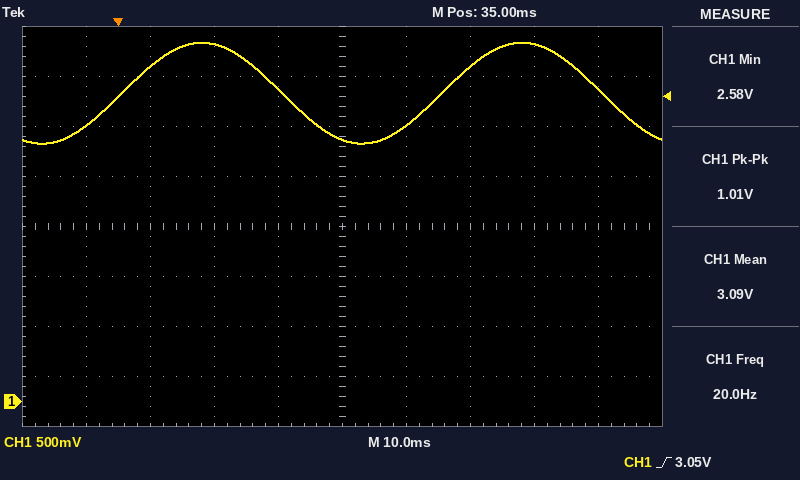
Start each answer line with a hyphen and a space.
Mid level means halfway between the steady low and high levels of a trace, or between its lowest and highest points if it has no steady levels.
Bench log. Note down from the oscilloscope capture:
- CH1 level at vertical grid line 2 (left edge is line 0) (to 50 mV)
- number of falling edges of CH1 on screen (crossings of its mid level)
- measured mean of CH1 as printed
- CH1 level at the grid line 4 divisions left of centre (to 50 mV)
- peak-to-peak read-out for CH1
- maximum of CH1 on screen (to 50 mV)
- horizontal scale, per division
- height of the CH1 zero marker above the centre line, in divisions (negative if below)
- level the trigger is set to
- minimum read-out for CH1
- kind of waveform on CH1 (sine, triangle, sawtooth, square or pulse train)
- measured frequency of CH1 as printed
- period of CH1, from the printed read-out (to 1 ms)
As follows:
- 3.35 V
- 2
- 3.09 V
- 2.75 V
- 1.01 V
- 3.60 V
- 10 ms
- -3.5 div
- 3.05 V
- 2.58 V
- sine
- 20.0 Hz
- 50 ms
